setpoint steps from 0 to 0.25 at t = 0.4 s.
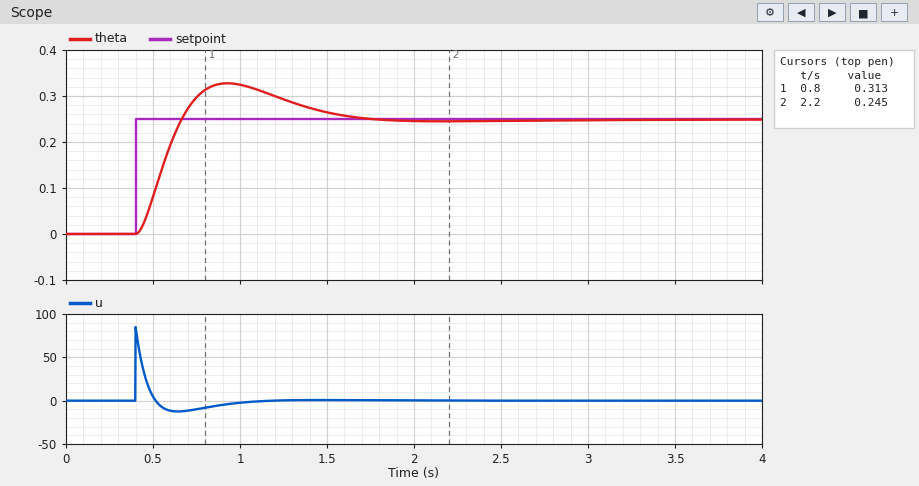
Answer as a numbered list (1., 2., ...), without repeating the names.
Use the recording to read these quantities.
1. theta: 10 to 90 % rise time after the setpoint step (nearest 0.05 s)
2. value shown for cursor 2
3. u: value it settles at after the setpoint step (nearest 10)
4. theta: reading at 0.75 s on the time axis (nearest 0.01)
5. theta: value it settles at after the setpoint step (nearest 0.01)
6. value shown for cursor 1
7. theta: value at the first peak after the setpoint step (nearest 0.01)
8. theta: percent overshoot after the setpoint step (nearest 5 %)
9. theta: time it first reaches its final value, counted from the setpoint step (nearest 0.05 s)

1. 0.20 s
2. 0.245
3. 0
4. 0.30
5. 0.25
6. 0.313
7. 0.33
8. 30 %
9. 0.25 s
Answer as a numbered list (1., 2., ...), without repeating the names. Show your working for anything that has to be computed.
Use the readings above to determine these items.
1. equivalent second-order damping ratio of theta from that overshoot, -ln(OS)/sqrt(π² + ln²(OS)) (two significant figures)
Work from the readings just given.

1. ln(0.3) = -1.204; 1.204 / sqrt(9.870 + 1.450) = 0.36
